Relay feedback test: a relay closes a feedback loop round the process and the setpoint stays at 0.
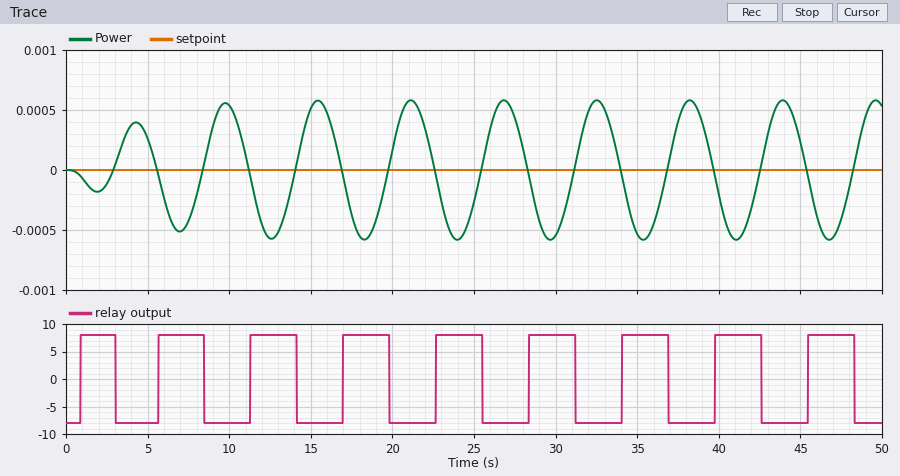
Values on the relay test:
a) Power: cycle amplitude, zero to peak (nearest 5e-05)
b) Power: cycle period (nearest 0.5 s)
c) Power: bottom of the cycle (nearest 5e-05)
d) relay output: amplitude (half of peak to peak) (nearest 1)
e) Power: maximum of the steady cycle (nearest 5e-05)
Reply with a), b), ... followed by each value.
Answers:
a) 0.00060
b) 5.5 s
c) -0.00060
d) 8
e) 0.00060
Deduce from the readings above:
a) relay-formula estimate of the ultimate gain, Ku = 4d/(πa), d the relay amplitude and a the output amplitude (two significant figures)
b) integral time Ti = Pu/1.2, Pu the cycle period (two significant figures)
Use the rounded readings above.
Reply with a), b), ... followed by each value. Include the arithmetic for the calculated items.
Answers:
a) 4 × 8 / (π × 0.0006) = 17000
b) 5.5 / 1.2 = 4.6 s
